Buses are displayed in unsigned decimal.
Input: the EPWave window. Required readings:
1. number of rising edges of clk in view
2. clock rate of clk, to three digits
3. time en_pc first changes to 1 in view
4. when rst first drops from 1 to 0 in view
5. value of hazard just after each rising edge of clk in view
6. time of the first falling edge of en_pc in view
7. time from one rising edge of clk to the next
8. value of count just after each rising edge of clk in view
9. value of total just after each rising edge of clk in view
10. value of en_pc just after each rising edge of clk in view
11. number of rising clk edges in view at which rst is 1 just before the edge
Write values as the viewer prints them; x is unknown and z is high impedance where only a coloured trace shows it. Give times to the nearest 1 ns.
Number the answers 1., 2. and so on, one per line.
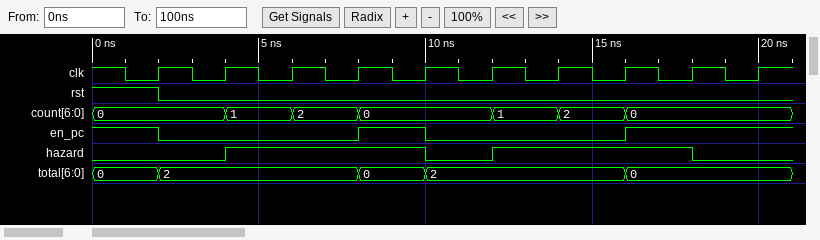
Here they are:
1. 10
2. 500 MHz
3. 8 ns
4. 2 ns
5. 0 1 1 1 0 1 1 1 0 0
6. 2 ns
7. 2 ns
8. 0, 1, 2, 0, 0, 1, 2, 0, 0, 0
9. 2, 2, 2, 0, 2, 2, 2, 0, 0, 0
10. 0 0 0 1 0 0 0 1 1 1
11. 1
